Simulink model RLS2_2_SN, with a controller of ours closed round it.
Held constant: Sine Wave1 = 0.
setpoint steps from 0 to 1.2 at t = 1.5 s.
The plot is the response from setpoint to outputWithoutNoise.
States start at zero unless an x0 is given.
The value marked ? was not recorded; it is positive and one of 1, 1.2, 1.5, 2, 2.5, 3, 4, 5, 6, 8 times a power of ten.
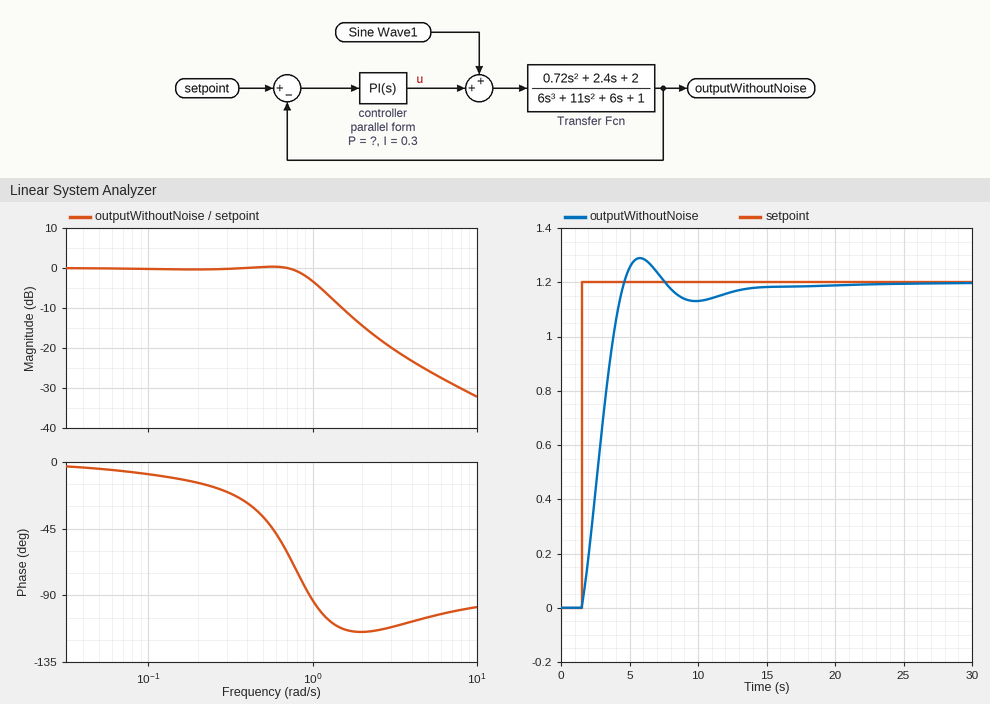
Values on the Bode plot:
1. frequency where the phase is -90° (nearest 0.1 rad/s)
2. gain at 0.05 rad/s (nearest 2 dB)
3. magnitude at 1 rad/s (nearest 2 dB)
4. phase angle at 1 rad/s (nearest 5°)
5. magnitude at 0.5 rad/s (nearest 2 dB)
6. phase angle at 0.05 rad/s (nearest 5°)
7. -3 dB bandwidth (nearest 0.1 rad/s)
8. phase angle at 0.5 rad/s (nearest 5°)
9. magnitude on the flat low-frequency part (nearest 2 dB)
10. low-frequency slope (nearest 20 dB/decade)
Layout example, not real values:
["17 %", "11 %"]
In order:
["1.0 rad/s", "0 dB", "-4 dB", "-95°", "0 dB", "-5°", "1.0 rad/s", "-35°", "0 dB", "0 dB/decade"]
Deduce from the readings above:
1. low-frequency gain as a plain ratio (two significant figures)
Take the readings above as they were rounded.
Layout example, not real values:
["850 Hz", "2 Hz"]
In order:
["1.0"]
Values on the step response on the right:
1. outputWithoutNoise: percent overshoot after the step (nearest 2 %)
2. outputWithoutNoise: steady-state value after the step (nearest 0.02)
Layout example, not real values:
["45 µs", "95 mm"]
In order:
["8 %", "1.20"]
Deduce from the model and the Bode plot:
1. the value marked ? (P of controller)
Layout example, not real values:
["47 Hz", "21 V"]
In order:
["2"]
